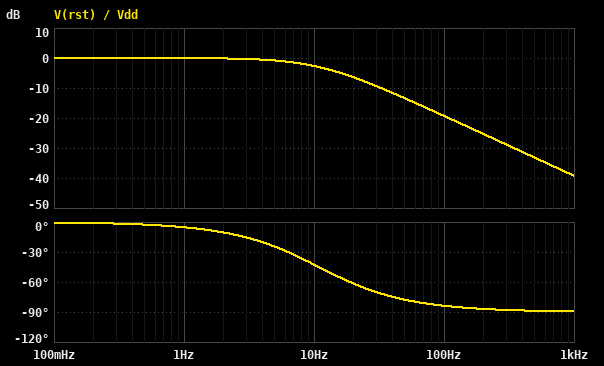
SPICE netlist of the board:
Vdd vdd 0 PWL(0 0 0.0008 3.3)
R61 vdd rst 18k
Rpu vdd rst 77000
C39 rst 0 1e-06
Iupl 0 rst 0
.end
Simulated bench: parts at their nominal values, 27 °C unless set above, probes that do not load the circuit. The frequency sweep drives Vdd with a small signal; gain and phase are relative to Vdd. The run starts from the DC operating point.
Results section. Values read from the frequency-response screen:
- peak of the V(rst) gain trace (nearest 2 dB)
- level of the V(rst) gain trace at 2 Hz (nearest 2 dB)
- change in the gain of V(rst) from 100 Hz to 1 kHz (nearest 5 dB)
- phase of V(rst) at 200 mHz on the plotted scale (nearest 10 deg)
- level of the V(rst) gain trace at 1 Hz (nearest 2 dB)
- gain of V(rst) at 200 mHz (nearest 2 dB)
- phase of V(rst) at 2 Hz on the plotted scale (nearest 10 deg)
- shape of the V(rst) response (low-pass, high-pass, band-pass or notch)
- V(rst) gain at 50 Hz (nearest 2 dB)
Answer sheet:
0 dB
0 dB
-20 dB
0 deg
0 dB
0 dB
-10 deg
low-pass
-14 dB
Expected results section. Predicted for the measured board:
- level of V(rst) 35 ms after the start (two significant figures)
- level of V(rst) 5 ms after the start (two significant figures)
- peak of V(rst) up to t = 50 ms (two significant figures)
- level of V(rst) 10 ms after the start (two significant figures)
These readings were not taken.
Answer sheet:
3.0 V
890 mV
3.2 V
1.6 V
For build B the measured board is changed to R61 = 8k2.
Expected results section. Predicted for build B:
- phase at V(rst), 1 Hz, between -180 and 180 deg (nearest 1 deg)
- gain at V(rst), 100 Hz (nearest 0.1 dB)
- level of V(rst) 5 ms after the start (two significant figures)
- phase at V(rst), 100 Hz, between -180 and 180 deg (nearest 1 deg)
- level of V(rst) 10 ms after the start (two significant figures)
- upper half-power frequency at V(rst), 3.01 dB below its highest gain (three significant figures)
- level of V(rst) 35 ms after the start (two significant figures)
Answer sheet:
-3 deg
-13.6 dB
1.5 V
-78 deg
2.4 V
21.5 Hz
3.3 V
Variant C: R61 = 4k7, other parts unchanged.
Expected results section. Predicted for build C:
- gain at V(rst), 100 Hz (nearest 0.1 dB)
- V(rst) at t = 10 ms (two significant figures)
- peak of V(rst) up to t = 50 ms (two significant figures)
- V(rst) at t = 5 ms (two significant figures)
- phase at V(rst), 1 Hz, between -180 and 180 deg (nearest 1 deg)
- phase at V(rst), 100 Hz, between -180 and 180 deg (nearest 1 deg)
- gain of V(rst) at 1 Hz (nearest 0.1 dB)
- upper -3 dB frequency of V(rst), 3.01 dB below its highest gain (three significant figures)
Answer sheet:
-9.4 dB
2.9 V
3.3 V
2.1 V
-2 deg
-70 deg
0 dB
35.9 Hz
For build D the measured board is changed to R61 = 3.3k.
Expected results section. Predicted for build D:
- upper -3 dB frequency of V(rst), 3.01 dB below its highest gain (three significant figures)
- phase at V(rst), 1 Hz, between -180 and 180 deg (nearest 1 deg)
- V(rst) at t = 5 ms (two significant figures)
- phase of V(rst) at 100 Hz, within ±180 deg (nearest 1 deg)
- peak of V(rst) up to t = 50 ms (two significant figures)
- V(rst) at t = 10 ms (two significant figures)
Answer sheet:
50.3 Hz
-1 deg
2.5 V
-63 deg
3.3 V
3.1 V
